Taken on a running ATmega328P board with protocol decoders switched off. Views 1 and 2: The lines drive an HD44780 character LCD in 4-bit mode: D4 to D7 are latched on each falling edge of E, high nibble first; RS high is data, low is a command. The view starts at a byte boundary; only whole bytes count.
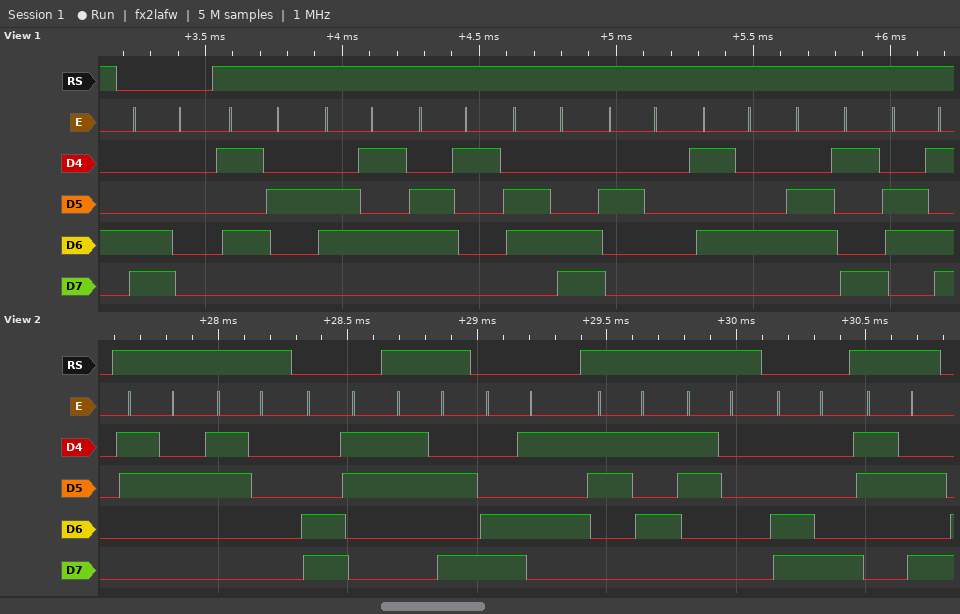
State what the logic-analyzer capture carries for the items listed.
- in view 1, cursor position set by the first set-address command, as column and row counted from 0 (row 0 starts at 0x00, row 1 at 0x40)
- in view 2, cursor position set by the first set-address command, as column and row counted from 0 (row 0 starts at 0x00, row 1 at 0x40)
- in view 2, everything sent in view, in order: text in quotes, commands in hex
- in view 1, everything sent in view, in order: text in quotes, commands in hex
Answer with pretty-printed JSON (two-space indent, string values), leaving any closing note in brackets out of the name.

{
  "in view 1, cursor position set by the first set-address command, as column and row counted from 0": "column 0, row 1",
  "in view 2, cursor position set by the first set-address command, as column and row counted from 0": "column 3, row 1",
  "in view 2, everything sent in view, in order: text in quotes, commands in hex": "\"20\" 0xC3 \":\" 0xC5 \"50\" 0xC8 \":\"",
  "in view 1, everything sent in view, in order: text in quotes, commands in hex": "0xC0 \"Real Tim\""
}
